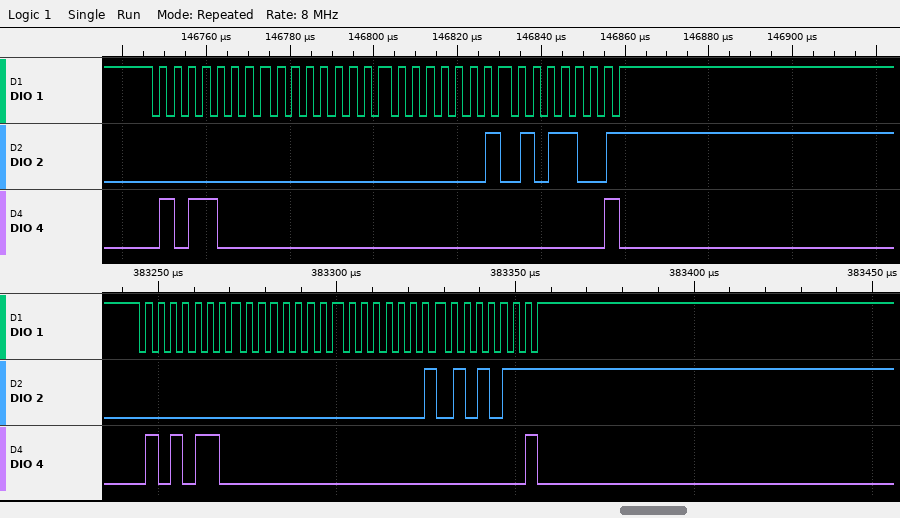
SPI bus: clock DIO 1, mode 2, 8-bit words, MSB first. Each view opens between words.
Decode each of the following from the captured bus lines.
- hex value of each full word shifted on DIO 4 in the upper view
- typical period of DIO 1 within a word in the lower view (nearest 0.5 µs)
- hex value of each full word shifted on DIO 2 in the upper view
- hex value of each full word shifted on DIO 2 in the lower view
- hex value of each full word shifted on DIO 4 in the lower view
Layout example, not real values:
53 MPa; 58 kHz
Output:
58, 00, 00, 01; 3.5 µs; 00, 00, 01, 59; 00, 00, 01, 57; 56, 00, 00, 01
